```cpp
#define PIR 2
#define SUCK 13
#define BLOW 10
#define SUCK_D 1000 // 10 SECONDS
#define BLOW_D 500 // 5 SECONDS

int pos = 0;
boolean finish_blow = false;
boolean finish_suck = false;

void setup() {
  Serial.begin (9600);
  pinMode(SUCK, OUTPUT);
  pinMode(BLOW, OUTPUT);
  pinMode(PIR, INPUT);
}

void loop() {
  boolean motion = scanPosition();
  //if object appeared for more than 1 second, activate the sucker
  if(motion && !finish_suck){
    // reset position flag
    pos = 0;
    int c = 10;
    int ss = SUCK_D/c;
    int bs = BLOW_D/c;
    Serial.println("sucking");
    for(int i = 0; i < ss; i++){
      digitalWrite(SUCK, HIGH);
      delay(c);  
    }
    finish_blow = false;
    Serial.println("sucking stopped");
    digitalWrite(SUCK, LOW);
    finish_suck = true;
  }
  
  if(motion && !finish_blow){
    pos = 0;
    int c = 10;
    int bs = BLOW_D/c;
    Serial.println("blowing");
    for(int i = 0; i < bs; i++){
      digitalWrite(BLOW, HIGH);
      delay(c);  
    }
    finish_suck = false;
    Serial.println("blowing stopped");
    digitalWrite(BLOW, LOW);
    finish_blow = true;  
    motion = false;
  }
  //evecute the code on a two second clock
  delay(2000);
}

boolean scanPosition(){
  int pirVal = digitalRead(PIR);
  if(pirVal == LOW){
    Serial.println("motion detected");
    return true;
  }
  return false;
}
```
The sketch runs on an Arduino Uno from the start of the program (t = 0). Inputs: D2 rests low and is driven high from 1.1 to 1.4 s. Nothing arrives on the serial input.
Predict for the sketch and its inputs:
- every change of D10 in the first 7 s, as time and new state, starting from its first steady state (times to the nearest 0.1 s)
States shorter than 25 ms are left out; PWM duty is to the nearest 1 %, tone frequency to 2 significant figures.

0 s low; 1 s high; 1.5 s low; 4.5 s high; 5 s low
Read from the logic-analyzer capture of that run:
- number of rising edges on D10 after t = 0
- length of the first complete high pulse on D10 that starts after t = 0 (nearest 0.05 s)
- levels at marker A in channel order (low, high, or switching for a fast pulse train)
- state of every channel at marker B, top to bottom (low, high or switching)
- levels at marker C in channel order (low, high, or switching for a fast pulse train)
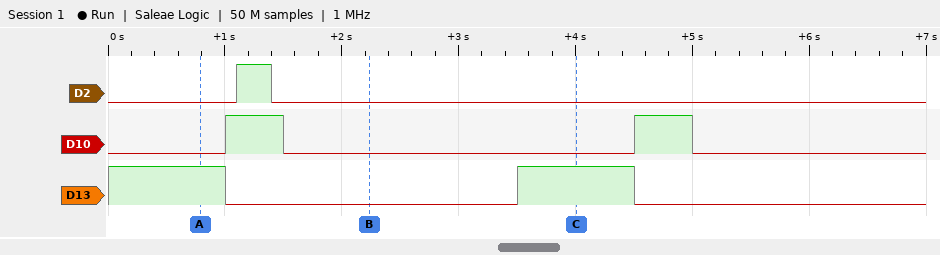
2
0.50 s
D2 low, D10 low, D13 high
D2 low, D10 low, D13 low
D2 low, D10 low, D13 high
